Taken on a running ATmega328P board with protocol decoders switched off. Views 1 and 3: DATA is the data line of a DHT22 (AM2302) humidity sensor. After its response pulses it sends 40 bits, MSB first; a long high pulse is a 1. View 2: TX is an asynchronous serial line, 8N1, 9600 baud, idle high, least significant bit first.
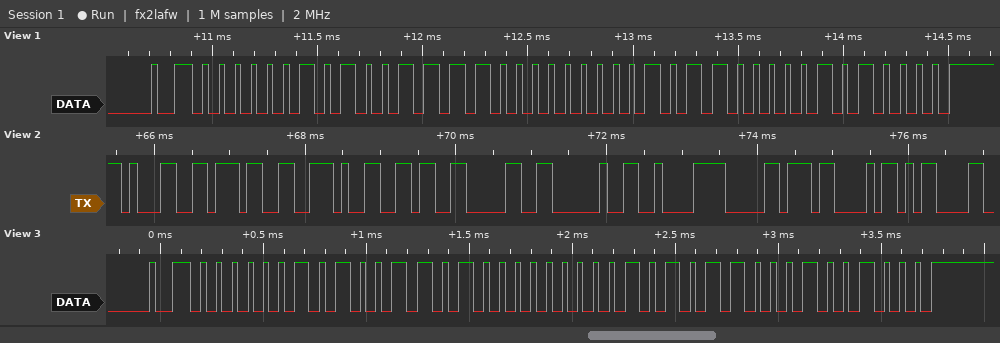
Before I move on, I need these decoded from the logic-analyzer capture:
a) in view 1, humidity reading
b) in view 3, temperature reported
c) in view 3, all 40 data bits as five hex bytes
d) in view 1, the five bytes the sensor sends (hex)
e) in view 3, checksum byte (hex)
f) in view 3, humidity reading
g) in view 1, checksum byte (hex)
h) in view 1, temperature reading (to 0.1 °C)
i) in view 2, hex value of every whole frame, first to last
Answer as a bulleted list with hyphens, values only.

- 67.0 %
- 17.2 °C
- 02 9A 00 AC 48
- 02 9E 00 B0 50
- 0x48
- 66.6 %
- 0x50
- 17.6 °C
- 0x31 0x37 0x2E 0x36 0x30 0x20 0xC2 0xB0 0x43 0x0D
